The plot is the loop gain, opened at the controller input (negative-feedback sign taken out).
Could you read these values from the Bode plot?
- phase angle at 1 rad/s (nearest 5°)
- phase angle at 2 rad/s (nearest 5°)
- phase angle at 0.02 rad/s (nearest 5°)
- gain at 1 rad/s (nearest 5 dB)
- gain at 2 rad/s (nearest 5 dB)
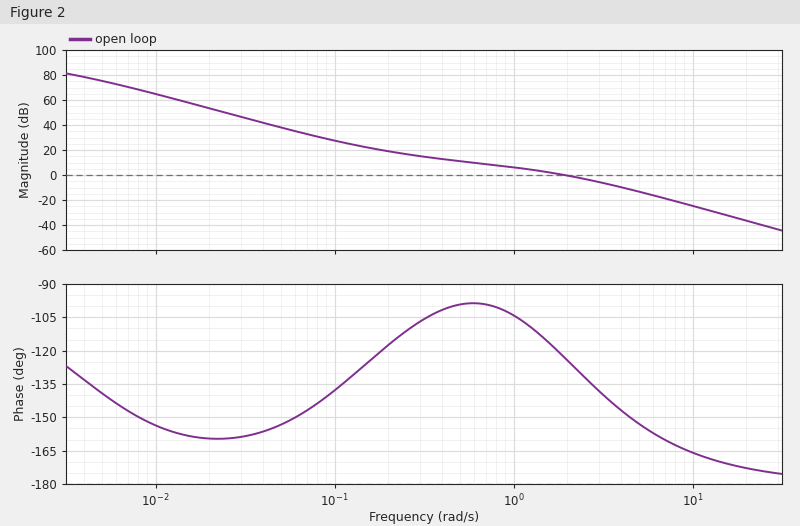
-105°
-125°
-160°
5 dB
0 dB
